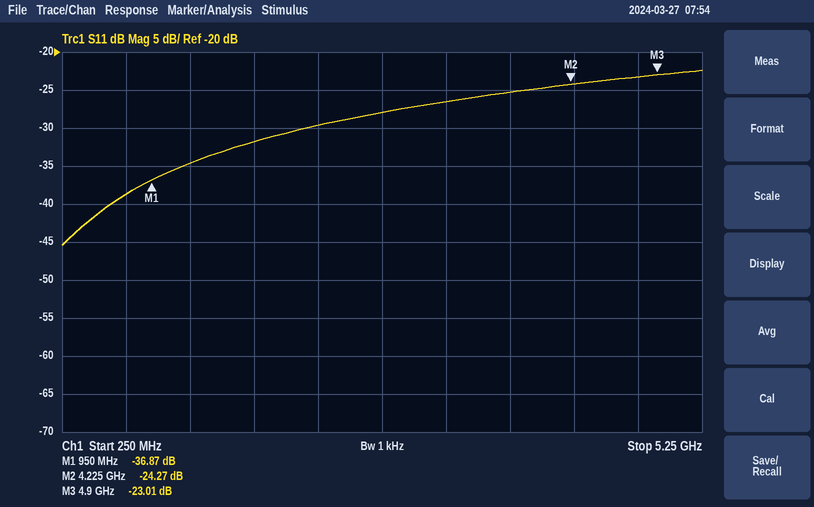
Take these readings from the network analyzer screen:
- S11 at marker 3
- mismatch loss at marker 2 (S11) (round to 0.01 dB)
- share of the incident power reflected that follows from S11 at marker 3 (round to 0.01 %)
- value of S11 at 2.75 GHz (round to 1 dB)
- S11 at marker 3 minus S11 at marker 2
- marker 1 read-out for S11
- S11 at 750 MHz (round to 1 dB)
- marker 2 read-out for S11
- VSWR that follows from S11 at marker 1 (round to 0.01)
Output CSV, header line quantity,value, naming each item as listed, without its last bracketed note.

quantity,value
S11 at marker 3,-23.01 dB
mismatch loss at marker 2 (S11),0.02 dB
share of the incident power reflected that follows from S11 at marker 3,0.50 %
value of S11 at 2.75 GHz,-28 dB
S11 at marker 3 minus S11 at marker 2,1.26 dB
marker 1 read-out for S11,-36.87 dB
S11 at 750 MHz,-39 dB
marker 2 read-out for S11,-24.27 dB
VSWR that follows from S11 at marker 1,1.03
